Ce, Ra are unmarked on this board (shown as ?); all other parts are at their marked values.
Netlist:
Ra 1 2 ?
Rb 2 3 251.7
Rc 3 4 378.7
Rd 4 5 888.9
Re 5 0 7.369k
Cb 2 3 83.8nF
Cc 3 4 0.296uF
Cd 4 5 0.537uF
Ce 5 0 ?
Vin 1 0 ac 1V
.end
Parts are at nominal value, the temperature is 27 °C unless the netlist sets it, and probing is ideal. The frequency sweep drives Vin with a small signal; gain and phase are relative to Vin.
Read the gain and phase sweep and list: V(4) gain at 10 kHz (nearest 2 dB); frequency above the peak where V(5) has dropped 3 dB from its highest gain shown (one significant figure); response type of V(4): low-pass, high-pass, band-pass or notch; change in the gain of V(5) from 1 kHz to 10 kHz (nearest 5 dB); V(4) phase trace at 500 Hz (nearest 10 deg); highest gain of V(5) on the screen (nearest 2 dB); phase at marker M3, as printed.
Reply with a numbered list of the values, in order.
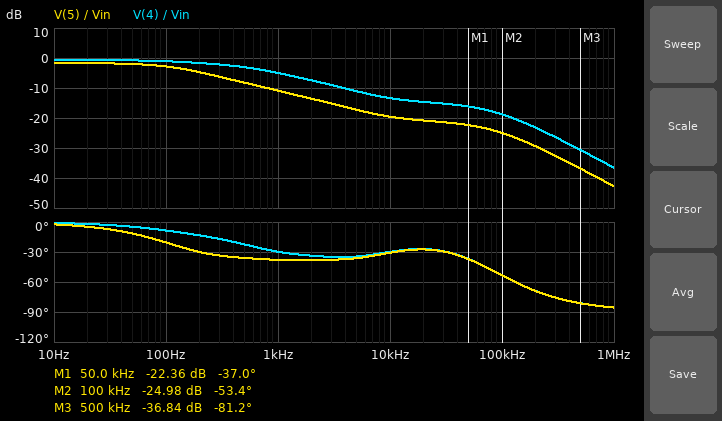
1. -14 dB
2. 200 Hz
3. low-pass
4. -10 dB
5. -20 deg
6. -2 dB
7. -81.2 deg
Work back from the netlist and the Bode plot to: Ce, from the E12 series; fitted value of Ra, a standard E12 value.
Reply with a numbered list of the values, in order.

1. 560 nF
2. 39 Ω
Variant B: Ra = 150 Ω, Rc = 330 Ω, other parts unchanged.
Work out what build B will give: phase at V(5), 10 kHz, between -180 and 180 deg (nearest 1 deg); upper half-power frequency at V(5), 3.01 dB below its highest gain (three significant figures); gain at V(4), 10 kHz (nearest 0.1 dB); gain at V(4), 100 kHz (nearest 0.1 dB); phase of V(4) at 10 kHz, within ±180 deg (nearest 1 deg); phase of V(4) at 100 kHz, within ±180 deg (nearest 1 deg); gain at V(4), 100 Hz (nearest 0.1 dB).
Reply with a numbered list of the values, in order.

1. -47 deg
2. 193 Hz
3. -15.4 dB
4. -28.5 dB
5. -46 deg
6. -79 deg
7. -1.2 dB
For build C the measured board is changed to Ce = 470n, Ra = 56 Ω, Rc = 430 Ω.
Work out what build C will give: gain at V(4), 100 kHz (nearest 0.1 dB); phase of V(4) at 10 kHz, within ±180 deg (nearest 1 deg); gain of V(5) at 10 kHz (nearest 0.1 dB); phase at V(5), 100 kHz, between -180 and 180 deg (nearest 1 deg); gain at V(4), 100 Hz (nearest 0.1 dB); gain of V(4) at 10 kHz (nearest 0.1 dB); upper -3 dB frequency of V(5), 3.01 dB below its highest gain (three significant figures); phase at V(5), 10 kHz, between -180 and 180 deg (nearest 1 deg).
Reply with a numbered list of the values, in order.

1. -20.2 dB
2. -32 deg
3. -18.5 dB
4. -62 deg
5. -1.1 dB
6. -13.0 dB
7. 228 Hz
8. -33 deg
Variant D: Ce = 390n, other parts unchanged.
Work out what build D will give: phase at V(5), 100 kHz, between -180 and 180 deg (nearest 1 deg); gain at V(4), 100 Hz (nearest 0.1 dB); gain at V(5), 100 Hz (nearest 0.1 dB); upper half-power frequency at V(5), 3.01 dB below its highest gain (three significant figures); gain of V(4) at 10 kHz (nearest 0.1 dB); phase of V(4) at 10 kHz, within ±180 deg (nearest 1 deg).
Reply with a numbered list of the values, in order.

1. -52 deg
2. -0.9 dB
3. -2.3 dB
4. 294 Hz
5. -12.0 dB
6. -29 deg
